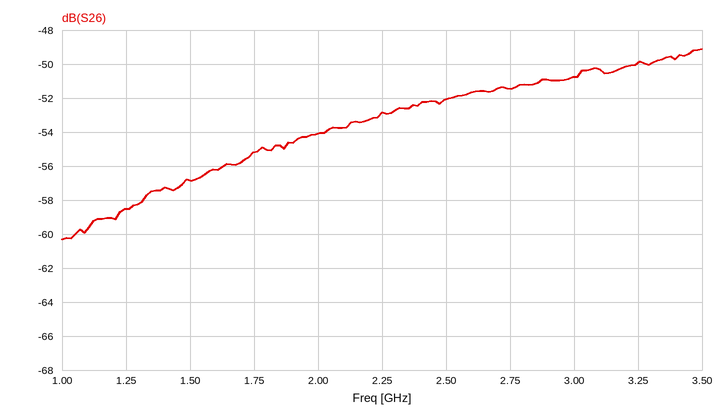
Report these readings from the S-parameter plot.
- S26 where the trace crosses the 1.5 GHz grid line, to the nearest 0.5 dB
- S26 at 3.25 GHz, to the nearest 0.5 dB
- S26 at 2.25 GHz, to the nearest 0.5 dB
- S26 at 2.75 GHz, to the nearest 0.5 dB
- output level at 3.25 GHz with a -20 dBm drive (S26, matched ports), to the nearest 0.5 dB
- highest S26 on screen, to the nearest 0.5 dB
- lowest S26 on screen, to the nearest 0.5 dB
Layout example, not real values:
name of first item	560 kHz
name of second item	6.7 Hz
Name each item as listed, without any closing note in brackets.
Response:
S26 where the trace crosses the 1.5 GHz grid line, to the nearest 0.5 dB	-57.0 dB
S26 at 3.25 GHz, to the nearest 0.5 dB	-50.0 dB
S26 at 2.25 GHz, to the nearest 0.5 dB	-53.0 dB
S26 at 2.75 GHz, to the nearest 0.5 dB	-51.5 dB
output level at 3.25 GHz with a -20 dBm drive (S26, matched ports), to the nearest 0.5 dB	-70.0 dBm
highest S26 on screen, to the nearest 0.5 dB	-49.0 dB
lowest S26 on screen, to the nearest 0.5 dB	-60.5 dB
